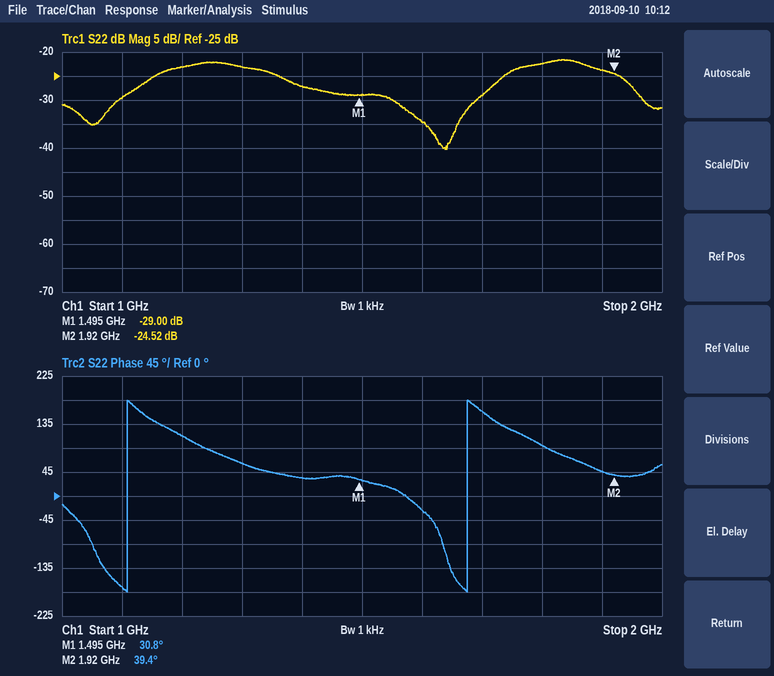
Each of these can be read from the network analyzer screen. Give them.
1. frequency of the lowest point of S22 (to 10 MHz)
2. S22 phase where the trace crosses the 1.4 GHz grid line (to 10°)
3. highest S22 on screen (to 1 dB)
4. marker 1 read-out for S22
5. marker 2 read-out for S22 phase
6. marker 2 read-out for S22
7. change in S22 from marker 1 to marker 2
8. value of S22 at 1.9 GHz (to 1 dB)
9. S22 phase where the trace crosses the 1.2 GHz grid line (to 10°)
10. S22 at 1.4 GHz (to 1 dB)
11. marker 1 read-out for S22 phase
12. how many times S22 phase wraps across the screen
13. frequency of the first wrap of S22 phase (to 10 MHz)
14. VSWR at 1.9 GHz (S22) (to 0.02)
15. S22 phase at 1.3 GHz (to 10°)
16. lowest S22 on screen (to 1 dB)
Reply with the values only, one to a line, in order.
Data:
1.64 GHz
30°
-22 dB
-29.00 dB
39.4°
-24.52 dB
4.48 dB
-24 dB
110°
-27 dB
30.8°
2
1.11 GHz
1.14
60°
-40 dB
